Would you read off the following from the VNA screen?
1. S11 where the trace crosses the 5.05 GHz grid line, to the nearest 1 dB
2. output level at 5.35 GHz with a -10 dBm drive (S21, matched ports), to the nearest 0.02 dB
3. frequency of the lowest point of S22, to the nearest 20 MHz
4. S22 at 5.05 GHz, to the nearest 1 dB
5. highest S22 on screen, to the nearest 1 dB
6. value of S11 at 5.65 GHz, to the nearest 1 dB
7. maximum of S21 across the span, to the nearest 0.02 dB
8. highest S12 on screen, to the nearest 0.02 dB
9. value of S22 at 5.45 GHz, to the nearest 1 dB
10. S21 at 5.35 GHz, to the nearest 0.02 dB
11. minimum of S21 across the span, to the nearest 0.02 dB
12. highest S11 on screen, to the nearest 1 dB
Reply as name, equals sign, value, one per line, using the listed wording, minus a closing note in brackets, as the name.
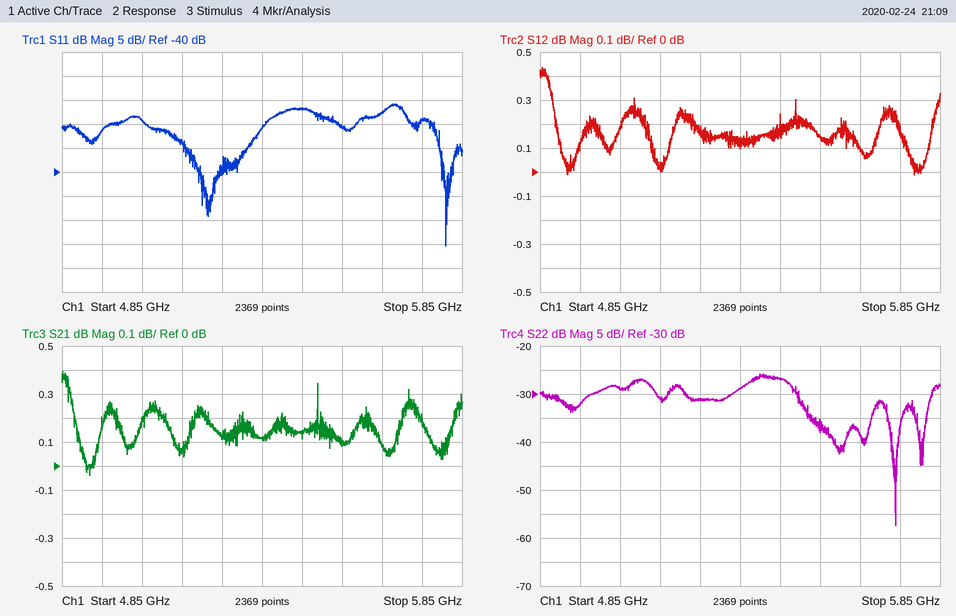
S11 where the trace crosses the 5.05 GHz grid line, to the nearest 1 dB = -29 dB
output level at 5.35 GHz with a -10 dBm drive (S21, matched ports), to the nearest 0.02 dB = -9.88 dBm
frequency of the lowest point of S22, to the nearest 20 MHz = 5.74 GHz
S22 at 5.05 GHz, to the nearest 1 dB = -29 dB
highest S22 on screen, to the nearest 1 dB = -26 dB
value of S11 at 5.65 GHz, to the nearest 1 dB = -28 dB
maximum of S21 across the span, to the nearest 0.02 dB = 0.40 dB
highest S12 on screen, to the nearest 0.02 dB = 0.44 dB
value of S22 at 5.45 GHz, to the nearest 1 dB = -27 dB
S21 at 5.35 GHz, to the nearest 0.02 dB = 0.12 dB
minimum of S21 across the span, to the nearest 0.02 dB = -0.04 dB
highest S11 on screen, to the nearest 1 dB = -26 dB
